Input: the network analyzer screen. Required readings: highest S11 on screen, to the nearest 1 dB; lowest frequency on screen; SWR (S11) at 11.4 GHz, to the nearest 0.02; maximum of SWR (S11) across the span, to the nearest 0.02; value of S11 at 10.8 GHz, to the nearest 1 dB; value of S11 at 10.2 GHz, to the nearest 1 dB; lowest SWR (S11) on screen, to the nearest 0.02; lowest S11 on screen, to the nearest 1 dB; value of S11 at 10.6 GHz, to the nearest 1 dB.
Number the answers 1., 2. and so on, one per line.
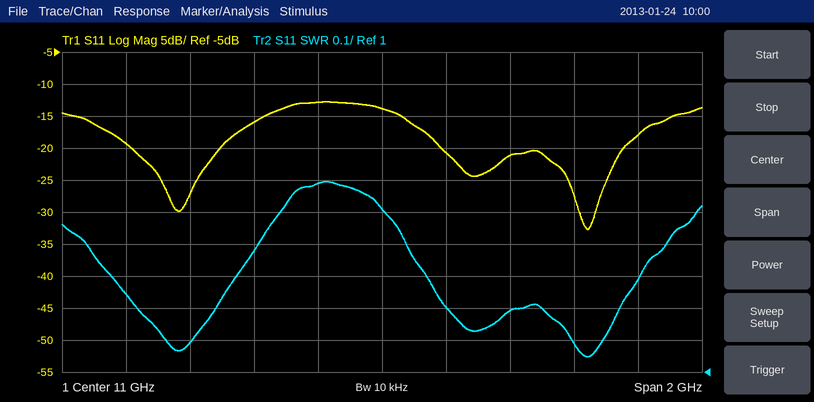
1. -13 dB
2. 10 GHz
3. 1.20
4. 1.60
5. -13 dB
6. -19 dB
7. 1.04
8. -33 dB
9. -16 dB
